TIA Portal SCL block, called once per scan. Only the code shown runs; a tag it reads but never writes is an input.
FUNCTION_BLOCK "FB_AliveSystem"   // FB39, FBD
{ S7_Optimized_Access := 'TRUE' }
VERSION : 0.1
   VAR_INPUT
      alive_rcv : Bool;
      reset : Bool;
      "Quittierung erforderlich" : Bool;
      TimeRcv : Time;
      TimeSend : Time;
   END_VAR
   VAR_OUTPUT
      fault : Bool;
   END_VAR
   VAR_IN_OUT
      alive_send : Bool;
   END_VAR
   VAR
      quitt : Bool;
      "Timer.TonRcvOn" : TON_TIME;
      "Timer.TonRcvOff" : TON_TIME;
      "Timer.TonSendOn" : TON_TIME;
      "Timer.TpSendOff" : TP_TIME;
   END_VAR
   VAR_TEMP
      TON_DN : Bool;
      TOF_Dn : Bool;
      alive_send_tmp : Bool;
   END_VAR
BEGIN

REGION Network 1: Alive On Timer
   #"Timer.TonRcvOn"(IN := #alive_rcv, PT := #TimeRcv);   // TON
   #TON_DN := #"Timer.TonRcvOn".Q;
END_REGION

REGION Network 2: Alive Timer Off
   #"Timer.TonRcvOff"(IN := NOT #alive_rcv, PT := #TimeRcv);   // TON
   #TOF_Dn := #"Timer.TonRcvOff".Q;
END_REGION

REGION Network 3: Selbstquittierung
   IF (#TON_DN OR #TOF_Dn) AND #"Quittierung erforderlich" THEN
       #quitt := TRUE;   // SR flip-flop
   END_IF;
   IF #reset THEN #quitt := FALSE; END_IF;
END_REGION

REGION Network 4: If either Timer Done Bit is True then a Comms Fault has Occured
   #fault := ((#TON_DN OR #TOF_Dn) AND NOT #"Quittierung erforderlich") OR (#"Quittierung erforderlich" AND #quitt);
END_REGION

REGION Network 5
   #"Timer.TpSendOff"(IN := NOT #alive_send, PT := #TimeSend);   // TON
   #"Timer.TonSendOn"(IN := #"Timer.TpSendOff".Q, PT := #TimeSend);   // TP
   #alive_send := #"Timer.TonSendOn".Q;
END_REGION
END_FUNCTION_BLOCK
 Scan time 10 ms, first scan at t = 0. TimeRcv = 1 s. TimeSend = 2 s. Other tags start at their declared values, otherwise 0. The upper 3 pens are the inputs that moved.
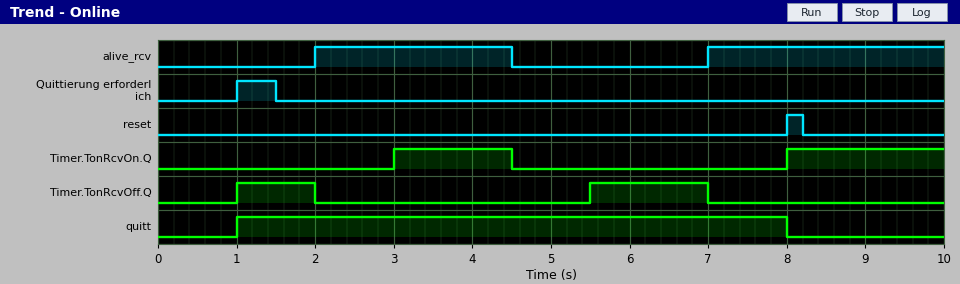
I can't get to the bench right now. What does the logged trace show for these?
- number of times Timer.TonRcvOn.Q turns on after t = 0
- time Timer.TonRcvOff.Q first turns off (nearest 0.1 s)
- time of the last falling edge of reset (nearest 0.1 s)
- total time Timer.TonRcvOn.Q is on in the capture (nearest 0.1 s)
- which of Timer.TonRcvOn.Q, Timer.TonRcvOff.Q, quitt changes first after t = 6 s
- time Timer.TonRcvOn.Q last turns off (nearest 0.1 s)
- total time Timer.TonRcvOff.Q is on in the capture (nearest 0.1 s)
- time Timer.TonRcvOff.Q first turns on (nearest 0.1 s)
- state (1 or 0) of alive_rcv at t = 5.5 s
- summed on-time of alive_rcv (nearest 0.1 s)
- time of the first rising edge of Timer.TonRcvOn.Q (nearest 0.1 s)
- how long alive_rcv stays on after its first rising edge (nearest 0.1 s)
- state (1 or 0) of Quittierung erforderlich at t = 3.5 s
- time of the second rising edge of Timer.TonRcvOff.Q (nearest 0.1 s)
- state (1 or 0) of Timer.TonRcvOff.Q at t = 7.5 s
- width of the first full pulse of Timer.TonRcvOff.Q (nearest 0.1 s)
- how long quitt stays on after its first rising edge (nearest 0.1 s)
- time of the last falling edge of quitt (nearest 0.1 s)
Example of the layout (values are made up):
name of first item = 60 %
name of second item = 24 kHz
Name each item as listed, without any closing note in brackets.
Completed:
number of times Timer.TonRcvOn.Q turns on after t = 0 = 2
time Timer.TonRcvOff.Q first turns off = 2.0 s
time of the last falling edge of reset = 8.2 s
total time Timer.TonRcvOn.Q is on in the capture = 3.5 s
which of Timer.TonRcvOn.Q, Timer.TonRcvOff.Q, quitt changes first after t = 6 s = Timer.TonRcvOff.Q
time Timer.TonRcvOn.Q last turns off = 4.5 s
total time Timer.TonRcvOff.Q is on in the capture = 2.5 s
time Timer.TonRcvOff.Q first turns on = 1.0 s
state (1 or 0) of alive_rcv at t = 5.5 s = 0
summed on-time of alive_rcv = 5.5 s
time of the first rising edge of Timer.TonRcvOn.Q = 3.0 s
how long alive_rcv stays on after its first rising edge = 2.5 s
state (1 or 0) of Quittierung erforderlich at t = 3.5 s = 0
time of the second rising edge of Timer.TonRcvOff.Q = 5.5 s
state (1 or 0) of Timer.TonRcvOff.Q at t = 7.5 s = 0
width of the first full pulse of Timer.TonRcvOff.Q = 1.0 s
how long quitt stays on after its first rising edge = 7.0 s
time of the last falling edge of quitt = 8.0 s
